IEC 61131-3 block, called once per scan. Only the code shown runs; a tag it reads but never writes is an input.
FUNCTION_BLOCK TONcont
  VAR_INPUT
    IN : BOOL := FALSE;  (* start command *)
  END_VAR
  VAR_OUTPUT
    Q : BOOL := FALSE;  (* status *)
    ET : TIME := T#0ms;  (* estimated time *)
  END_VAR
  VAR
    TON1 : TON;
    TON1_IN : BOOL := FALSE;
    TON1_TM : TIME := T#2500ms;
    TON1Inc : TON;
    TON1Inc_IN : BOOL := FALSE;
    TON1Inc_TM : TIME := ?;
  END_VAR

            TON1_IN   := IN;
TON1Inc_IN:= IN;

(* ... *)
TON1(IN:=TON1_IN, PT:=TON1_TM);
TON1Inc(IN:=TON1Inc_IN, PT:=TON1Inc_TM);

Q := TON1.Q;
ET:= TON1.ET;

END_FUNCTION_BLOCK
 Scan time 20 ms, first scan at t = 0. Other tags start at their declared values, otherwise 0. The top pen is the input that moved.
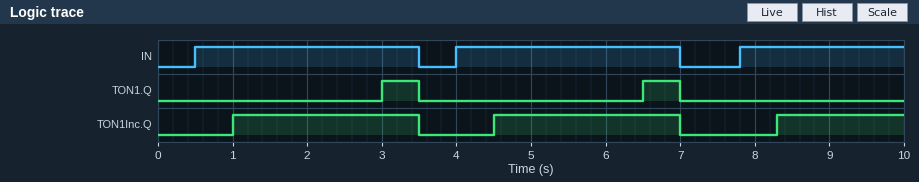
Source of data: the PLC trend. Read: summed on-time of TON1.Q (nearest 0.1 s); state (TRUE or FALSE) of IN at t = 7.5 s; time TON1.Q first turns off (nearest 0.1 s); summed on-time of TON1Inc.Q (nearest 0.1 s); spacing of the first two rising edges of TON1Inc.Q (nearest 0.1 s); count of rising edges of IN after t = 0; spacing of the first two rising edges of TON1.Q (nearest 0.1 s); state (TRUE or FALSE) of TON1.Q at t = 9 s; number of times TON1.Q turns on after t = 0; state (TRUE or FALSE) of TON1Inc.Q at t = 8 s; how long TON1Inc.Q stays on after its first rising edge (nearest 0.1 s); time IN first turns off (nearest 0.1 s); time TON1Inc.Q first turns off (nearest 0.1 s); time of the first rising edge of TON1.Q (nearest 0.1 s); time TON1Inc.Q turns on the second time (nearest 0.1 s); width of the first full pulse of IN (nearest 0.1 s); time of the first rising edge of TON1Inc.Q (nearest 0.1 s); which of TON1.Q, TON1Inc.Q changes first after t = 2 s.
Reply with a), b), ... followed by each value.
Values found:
a) 1.0 s
b) FALSE
c) 3.5 s
d) 6.7 s
e) 3.5 s
f) 3
g) 3.5 s
h) FALSE
i) 2
j) FALSE
k) 2.5 s
l) 3.5 s
m) 3.5 s
n) 3.0 s
o) 4.5 s
p) 3.0 s
q) 1.0 s
r) TON1.Q
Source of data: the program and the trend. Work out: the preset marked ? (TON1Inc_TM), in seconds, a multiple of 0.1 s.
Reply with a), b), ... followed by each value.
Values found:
a) 0.5 s
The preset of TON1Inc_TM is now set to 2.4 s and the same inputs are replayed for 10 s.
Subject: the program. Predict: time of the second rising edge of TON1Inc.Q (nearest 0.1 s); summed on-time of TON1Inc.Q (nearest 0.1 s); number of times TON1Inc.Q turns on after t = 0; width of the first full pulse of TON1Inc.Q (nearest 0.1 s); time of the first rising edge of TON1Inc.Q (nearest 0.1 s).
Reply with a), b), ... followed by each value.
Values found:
a) 6.4 s
b) 1.2 s
c) 2
d) 0.6 s
e) 2.9 s
